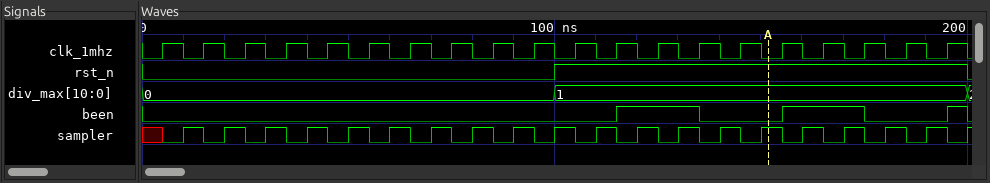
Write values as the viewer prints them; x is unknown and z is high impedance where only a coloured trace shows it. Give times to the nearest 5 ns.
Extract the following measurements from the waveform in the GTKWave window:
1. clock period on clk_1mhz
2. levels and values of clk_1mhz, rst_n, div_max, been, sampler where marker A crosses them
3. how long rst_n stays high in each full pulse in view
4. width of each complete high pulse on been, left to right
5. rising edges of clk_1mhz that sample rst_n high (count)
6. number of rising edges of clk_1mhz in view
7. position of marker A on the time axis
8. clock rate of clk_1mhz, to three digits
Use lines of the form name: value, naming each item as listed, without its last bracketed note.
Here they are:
clock period on clk_1mhz: 10 ns
levels and values of clk_1mhz, rst_n, div_max, been, sampler where marker A crosses them: clk_1mhz=0, rst_n=1, div_max=1, been=0, sampler=1
how long rst_n stays high in each full pulse in view: 100 ns
width of each complete high pulse on been, left to right: 20 ns, 20 ns, 5 ns
rising edges of clk_1mhz that sample rst_n high: 10
number of rising edges of clk_1mhz in view: 20
position of marker A on the time axis: 150 ns
clock rate of clk_1mhz, to three digits: 100 MHz
